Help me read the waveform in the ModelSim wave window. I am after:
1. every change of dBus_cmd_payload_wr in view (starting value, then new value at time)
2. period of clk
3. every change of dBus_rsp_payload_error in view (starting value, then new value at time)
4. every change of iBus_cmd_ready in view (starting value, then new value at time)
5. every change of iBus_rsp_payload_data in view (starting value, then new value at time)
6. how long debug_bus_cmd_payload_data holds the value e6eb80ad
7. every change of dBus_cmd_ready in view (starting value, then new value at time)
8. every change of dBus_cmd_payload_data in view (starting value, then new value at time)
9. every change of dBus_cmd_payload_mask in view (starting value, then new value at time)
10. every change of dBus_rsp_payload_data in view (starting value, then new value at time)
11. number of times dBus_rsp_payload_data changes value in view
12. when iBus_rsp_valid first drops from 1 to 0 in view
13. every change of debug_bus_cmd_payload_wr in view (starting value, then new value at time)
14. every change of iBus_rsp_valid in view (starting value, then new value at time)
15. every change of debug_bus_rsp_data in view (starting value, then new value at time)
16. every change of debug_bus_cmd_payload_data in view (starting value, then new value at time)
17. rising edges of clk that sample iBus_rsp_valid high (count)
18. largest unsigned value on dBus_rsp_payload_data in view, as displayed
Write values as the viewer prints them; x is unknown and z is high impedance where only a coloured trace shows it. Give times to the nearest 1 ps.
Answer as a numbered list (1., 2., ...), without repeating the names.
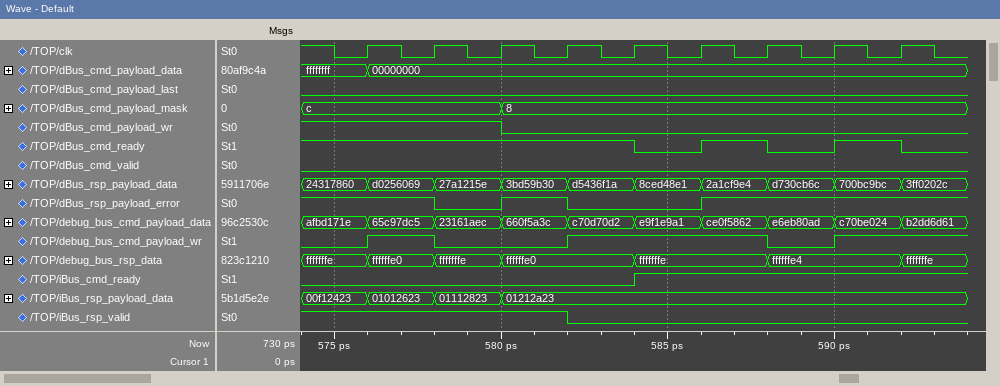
1. 1, 0 at 580 ps
2. 2 ps
3. 1, 0 at 578 ps, 1 at 580 ps, 0 at 582 ps, 1 at 586 ps
4. 0, 1 at 584 ps
5. 00f12423, 01012623 at 576 ps, 01112823 at 578 ps, 01212a23 at 580 ps
6. 2 ps
7. 1, 0 at 584 ps, 1 at 586 ps, 0 at 588 ps, 1 at 590 ps, 0 at 592 ps
8. ffffffff, 00000000 at 576 ps
9. c, 8 at 580 ps
10. 24317860, d0256069 at 576 ps, 27a1215e at 578 ps, 3bd59b30 at 580 ps, d5436f1a at 582 ps, 8ced48e1 at 584 ps, 2a1cf9e4 at 586 ps, d730cb6c at 588 ps, 700bc9bc at 590 ps, 3ff0202c at 592 ps
11. 9
12. 582 ps
13. 0, 1 at 576 ps, 0 at 578 ps, 1 at 582 ps, 0 at 588 ps, 1 at 590 ps
14. 1, 0 at 582 ps
15. fffffffe, ffffffe0 at 576 ps, fffffffe at 578 ps, ffffffe0 at 580 ps, fffffffe at 584 ps, ffffffe4 at 588 ps, fffffffe at 592 ps
16. afbd171e, 65c97dc5 at 576 ps, 23161aec at 578 ps, 660f5a3c at 580 ps, c70d70d2 at 582 ps, e9f1e9a1 at 584 ps, ce0f5862 at 586 ps, e6eb80ad at 588 ps, c70be024 at 590 ps, b2dd6d61 at 592 ps
17. 4
18. d730cb6c
